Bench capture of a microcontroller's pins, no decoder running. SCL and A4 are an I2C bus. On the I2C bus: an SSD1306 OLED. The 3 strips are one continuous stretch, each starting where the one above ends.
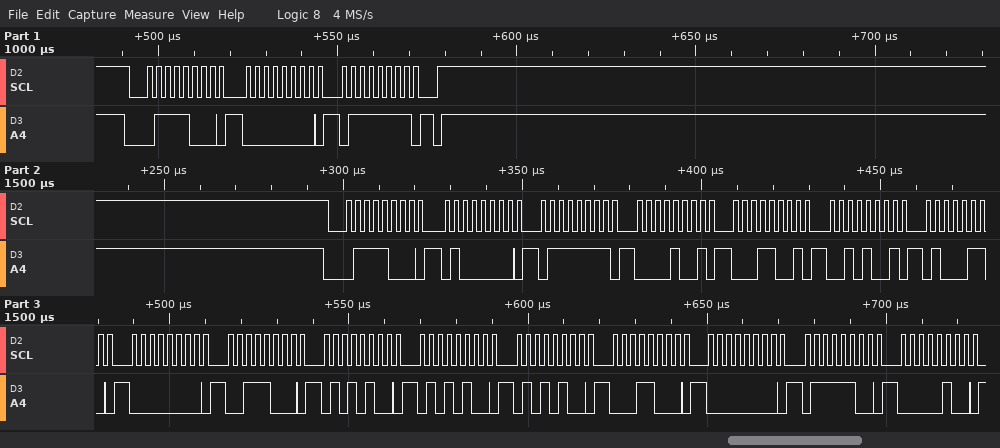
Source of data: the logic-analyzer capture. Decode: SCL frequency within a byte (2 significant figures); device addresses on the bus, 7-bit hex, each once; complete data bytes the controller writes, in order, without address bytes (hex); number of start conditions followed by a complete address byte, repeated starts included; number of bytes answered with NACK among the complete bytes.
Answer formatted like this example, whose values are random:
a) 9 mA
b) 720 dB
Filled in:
a) 400 kHz
b) 0x3C
c) 00 7F 40 7F 09 19 29 46 00 38 54 54 54 18 00 7C 04
d) 2
e) 0
